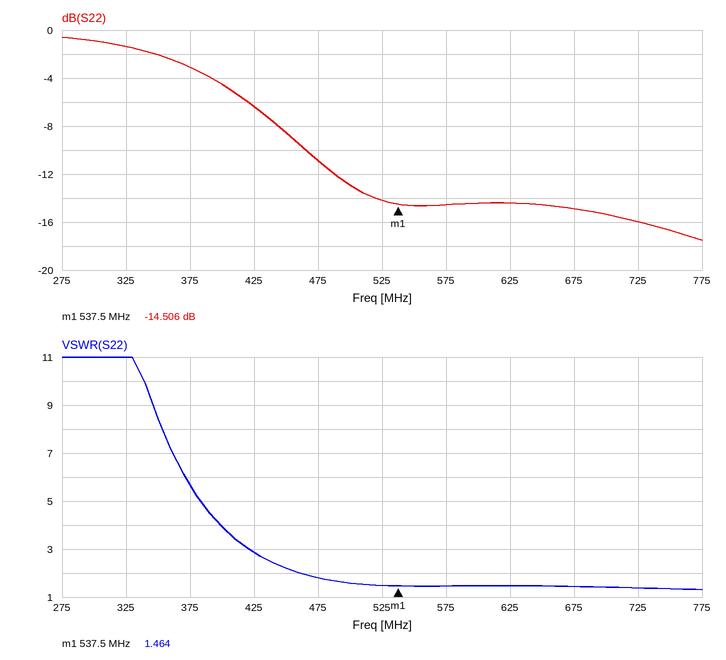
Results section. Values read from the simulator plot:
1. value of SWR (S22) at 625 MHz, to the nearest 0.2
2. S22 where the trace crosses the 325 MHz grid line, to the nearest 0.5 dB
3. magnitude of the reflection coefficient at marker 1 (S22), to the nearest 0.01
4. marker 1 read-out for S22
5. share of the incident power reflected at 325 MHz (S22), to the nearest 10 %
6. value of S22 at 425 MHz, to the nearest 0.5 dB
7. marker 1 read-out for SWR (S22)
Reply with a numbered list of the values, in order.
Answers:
1. 1.4
2. -1.5 dB
3. 0.19
4. -14.506 dB
5. 70 %
6. -6.5 dB
7. 1.464
